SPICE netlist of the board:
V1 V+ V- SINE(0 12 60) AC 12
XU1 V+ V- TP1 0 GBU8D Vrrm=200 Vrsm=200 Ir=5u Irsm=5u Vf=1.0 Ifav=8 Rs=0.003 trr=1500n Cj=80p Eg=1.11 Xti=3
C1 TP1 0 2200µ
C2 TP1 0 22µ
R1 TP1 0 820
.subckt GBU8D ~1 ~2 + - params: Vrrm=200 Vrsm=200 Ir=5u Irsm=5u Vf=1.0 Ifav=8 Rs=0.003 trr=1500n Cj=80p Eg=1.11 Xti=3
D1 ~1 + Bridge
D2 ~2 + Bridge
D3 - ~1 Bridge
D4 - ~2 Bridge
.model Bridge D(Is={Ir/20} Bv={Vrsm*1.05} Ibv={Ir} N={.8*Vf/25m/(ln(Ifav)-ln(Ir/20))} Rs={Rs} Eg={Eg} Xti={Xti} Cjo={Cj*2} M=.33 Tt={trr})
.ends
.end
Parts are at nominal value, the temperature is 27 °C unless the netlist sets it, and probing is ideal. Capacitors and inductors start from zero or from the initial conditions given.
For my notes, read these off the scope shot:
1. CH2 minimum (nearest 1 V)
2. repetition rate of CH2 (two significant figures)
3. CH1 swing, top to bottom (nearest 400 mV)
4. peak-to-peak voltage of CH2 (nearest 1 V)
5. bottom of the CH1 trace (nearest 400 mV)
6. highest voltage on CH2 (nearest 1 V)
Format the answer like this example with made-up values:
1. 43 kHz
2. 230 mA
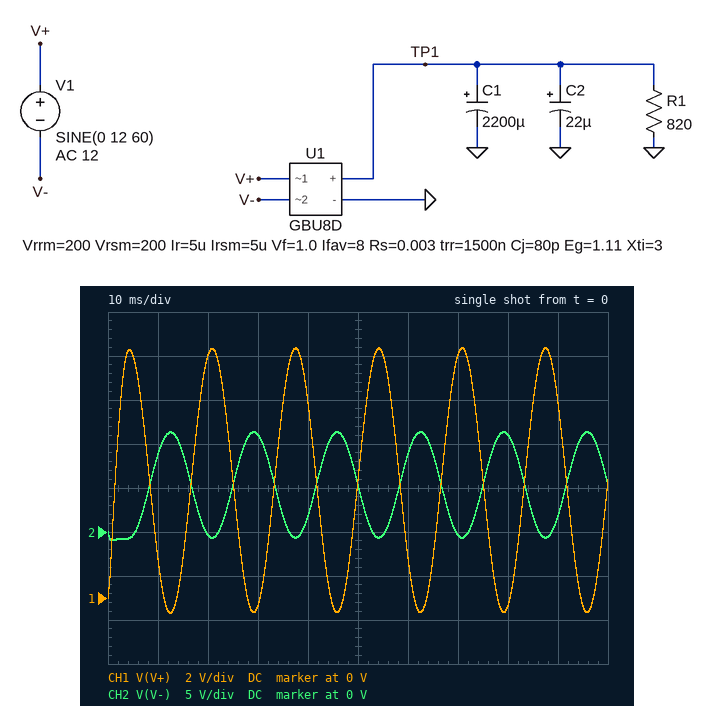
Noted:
1. -1 V
2. 60 Hz
3. 12.0 V
4. 12 V
5. -800 mV
6. 11 V
